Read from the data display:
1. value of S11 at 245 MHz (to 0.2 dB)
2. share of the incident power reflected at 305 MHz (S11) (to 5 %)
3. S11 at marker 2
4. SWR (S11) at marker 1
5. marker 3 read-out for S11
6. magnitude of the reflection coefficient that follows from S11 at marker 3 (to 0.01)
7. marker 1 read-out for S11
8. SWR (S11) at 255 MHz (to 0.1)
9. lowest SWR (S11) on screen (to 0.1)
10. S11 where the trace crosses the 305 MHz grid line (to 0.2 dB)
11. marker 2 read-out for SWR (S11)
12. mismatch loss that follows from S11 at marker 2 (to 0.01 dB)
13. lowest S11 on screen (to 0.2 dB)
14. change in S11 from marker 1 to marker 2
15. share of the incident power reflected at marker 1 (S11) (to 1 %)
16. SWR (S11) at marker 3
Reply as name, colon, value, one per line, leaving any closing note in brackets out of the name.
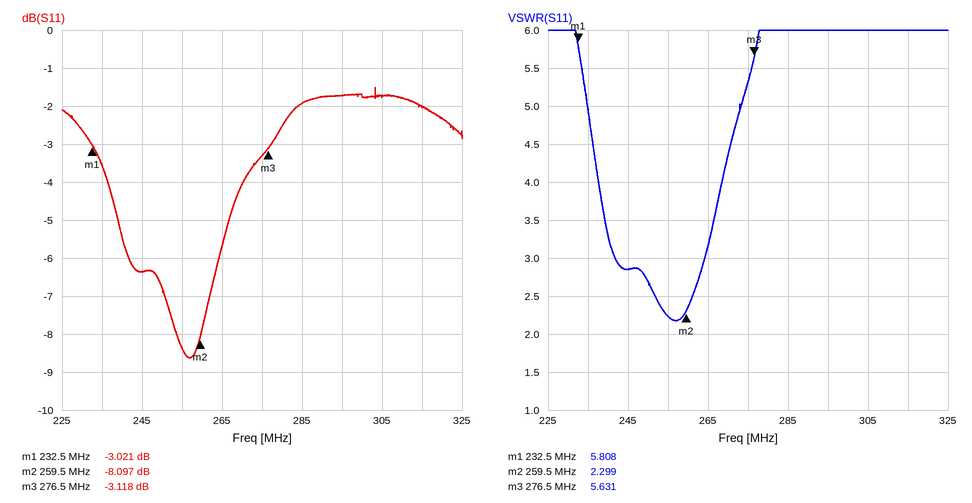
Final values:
value of S11 at 245 MHz: -6.4 dB
share of the incident power reflected at 305 MHz (S11): 65 %
S11 at marker 2: -8.097 dB
SWR (S11) at marker 1: 5.808
marker 3 read-out for S11: -3.118 dB
magnitude of the reflection coefficient that follows from S11 at marker 3: 0.70
marker 1 read-out for S11: -3.021 dB
SWR (S11) at 255 MHz: 2.2
lowest SWR (S11) on screen: 2.2
S11 where the trace crosses the 305 MHz grid line: -1.8 dB
marker 2 read-out for SWR: 2.299
mismatch loss that follows from S11 at marker 2: 0.73 dB
lowest S11 on screen: -8.6 dB
change in S11 from marker 1 to marker 2: -5.076 dB
share of the incident power reflected at marker 1 (S11): 50 %
SWR (S11) at marker 3: 5.631
